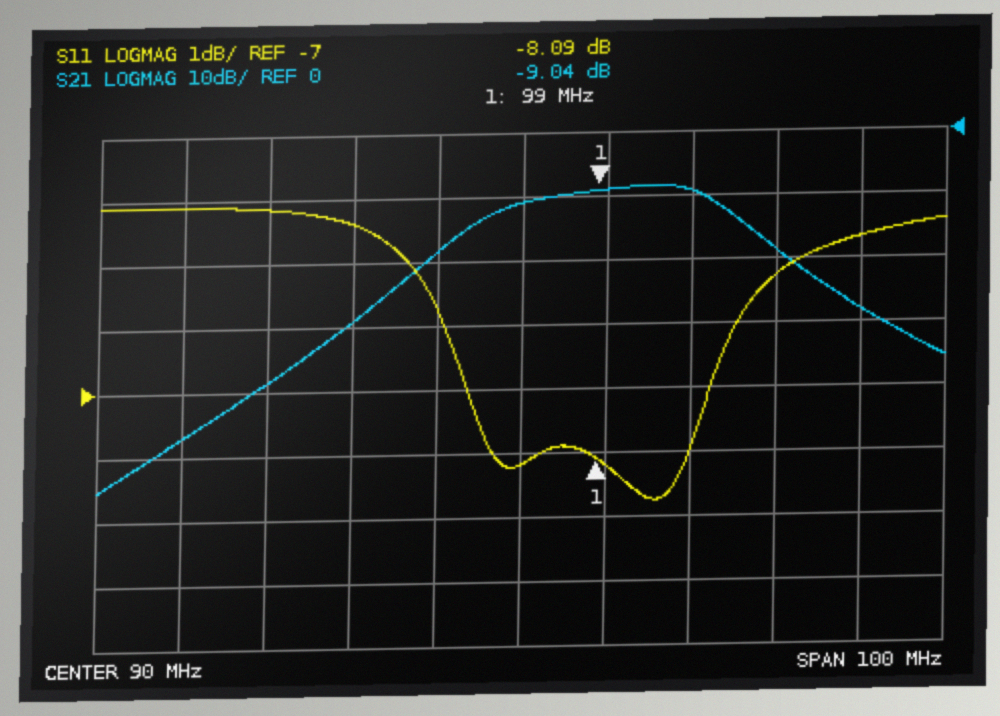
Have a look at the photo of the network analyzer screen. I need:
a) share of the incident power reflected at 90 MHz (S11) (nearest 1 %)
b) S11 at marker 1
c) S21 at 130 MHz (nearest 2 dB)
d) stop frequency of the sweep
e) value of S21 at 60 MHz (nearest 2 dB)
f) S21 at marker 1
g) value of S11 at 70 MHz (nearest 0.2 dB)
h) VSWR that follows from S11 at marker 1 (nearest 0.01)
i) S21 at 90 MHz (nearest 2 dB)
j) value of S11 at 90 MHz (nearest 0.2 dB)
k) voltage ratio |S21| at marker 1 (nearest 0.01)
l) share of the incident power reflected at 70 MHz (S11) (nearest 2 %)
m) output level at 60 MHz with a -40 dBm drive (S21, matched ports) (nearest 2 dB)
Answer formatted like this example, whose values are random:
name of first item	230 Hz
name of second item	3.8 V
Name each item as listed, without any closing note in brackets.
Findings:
share of the incident power reflected at 90 MHz (S11)	15 %
S11 at marker 1	-8.09 dB
S21 at 130 MHz	-28 dB
stop frequency of the sweep	140 MHz
value of S21 at 60 MHz	-38 dB
S21 at marker 1	-9.04 dB
value of S11 at 70 MHz	-4.4 dB
VSWR that follows from S11 at marker 1	2.30
S21 at 90 MHz	-10 dB
value of S11 at 90 MHz	-8.2 dB
voltage ratio |S21| at marker 1	0.35
share of the incident power reflected at 70 MHz (S11)	36 %
output level at 60 MHz with a -40 dBm drive (S21, matched ports)	-78 dBm
